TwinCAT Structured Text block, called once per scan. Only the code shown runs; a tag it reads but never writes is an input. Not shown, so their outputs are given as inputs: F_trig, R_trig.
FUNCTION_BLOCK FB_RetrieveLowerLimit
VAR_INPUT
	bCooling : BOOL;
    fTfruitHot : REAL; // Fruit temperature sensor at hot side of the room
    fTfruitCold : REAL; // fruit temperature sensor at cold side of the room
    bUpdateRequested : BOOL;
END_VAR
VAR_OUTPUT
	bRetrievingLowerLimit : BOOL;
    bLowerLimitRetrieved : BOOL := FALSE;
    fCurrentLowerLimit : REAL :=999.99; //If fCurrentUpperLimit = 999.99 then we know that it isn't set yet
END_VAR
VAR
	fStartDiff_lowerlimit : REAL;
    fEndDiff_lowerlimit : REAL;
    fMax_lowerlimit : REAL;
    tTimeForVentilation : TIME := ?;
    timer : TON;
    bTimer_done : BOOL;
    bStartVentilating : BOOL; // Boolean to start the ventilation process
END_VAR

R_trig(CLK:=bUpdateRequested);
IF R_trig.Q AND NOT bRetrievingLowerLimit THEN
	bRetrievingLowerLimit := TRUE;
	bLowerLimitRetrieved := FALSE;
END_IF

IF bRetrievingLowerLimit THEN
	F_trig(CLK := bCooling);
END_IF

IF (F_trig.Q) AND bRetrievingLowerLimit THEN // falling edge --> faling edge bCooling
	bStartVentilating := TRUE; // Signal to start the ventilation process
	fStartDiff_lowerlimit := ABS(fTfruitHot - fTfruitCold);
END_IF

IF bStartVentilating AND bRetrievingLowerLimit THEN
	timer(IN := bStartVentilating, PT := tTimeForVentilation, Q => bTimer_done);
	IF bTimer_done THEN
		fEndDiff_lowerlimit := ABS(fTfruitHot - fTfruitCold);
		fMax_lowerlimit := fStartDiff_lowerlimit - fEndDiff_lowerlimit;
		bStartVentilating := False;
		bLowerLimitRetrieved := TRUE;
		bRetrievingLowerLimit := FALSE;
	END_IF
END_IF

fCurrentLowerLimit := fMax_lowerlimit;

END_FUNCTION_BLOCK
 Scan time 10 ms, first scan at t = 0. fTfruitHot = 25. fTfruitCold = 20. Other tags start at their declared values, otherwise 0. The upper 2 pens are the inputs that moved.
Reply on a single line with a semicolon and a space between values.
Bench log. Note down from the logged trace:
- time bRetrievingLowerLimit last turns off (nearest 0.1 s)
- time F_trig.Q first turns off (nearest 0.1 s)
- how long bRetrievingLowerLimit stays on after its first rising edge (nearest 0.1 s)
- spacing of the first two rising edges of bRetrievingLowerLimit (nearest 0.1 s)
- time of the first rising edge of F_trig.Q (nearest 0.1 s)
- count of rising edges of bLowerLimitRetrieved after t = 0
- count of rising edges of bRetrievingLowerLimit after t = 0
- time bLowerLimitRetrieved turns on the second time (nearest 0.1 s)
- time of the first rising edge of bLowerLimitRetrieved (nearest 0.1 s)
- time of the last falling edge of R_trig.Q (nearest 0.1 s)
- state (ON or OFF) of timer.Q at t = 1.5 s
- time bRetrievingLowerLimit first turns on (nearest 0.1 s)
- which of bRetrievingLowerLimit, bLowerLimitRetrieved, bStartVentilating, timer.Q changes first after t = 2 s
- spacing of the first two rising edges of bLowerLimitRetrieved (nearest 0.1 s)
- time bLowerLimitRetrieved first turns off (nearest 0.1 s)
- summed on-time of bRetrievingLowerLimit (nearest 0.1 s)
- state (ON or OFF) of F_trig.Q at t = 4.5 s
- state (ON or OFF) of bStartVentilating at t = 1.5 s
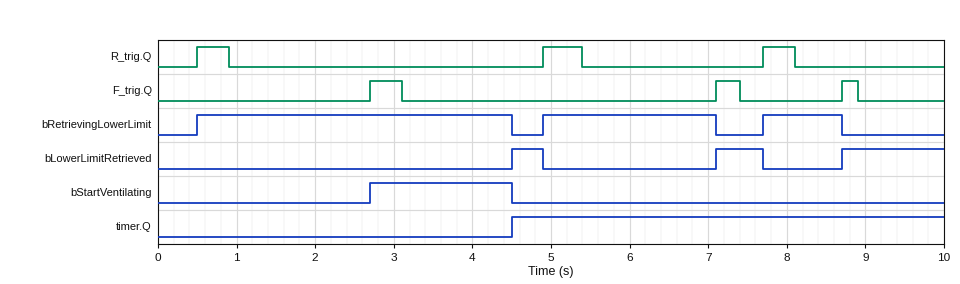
8.7 s; 3.1 s; 4.0 s; 4.4 s; 2.7 s; 3; 3; 7.1 s; 4.5 s; 8.1 s; OFF; 0.5 s; bStartVentilating; 2.6 s; 4.9 s; 7.2 s; OFF; OFF
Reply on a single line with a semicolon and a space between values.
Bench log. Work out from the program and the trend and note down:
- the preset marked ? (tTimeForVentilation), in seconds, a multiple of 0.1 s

1.8 s
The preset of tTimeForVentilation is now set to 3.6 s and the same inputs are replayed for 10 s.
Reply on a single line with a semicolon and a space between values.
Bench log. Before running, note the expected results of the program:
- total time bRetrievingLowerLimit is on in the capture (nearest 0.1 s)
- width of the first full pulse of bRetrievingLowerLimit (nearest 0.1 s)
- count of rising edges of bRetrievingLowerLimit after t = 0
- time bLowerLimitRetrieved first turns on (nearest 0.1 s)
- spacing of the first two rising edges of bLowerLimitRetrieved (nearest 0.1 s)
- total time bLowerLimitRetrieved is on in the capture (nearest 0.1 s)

6.8 s; 5.8 s; 2; 6.3 s; 2.4 s; 2.7 s
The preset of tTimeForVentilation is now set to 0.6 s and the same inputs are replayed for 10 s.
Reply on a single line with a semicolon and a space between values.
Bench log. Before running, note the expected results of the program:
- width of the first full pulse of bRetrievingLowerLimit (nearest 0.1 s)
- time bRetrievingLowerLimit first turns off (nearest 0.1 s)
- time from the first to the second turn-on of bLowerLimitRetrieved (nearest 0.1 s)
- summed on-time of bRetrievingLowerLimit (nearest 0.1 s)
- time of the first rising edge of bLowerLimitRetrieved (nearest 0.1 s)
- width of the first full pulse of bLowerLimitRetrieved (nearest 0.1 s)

2.8 s; 3.3 s; 3.8 s; 6.0 s; 3.3 s; 1.6 s
